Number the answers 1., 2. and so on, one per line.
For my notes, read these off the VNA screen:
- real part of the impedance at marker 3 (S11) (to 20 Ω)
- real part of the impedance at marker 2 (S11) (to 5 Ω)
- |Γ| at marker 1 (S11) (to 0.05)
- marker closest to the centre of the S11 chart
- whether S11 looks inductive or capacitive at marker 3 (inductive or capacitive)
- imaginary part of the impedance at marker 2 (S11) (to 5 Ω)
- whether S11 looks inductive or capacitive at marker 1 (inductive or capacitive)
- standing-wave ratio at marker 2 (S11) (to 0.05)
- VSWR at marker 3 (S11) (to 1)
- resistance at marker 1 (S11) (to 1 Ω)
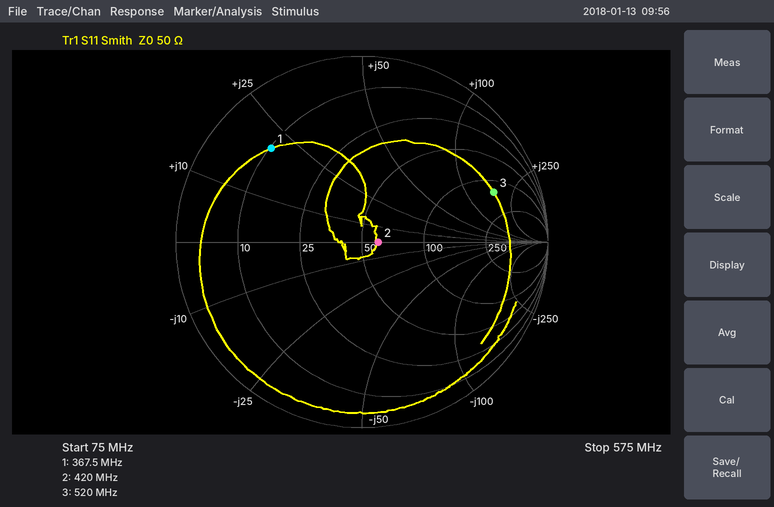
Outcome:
1. 140 Ω
2. 60 Ω
3. 0.70
4. marker 2
5. inductive
6. 0 Ω
7. inductive
8. 1.20
9. 7
10. 10 Ω
